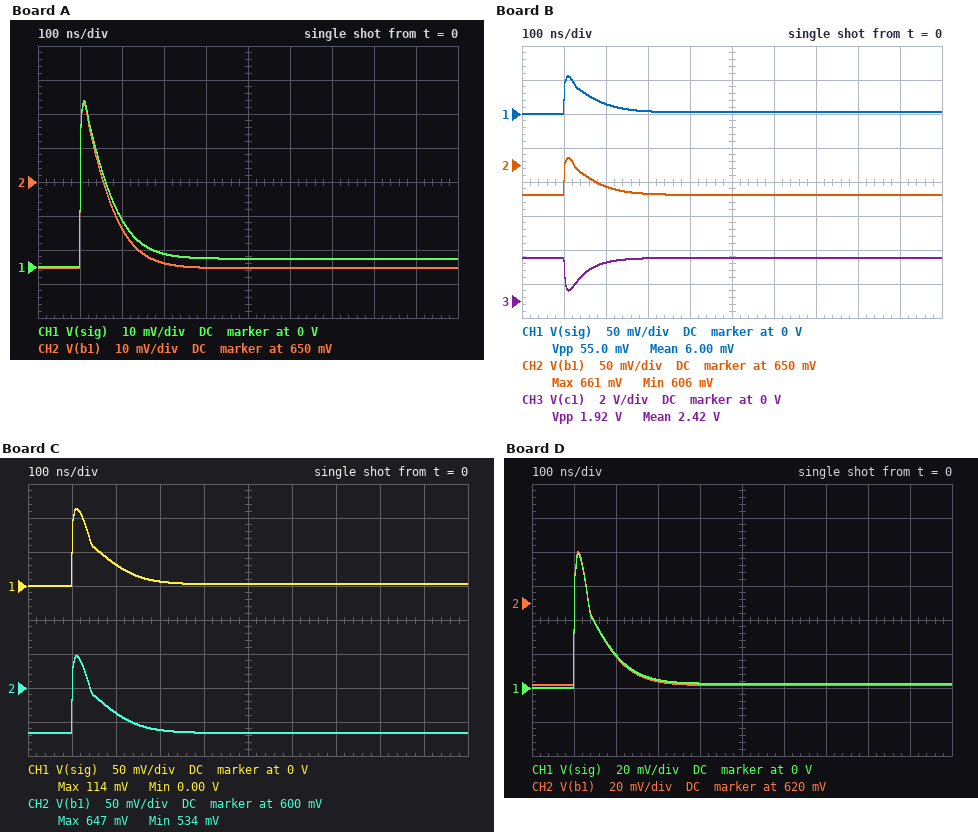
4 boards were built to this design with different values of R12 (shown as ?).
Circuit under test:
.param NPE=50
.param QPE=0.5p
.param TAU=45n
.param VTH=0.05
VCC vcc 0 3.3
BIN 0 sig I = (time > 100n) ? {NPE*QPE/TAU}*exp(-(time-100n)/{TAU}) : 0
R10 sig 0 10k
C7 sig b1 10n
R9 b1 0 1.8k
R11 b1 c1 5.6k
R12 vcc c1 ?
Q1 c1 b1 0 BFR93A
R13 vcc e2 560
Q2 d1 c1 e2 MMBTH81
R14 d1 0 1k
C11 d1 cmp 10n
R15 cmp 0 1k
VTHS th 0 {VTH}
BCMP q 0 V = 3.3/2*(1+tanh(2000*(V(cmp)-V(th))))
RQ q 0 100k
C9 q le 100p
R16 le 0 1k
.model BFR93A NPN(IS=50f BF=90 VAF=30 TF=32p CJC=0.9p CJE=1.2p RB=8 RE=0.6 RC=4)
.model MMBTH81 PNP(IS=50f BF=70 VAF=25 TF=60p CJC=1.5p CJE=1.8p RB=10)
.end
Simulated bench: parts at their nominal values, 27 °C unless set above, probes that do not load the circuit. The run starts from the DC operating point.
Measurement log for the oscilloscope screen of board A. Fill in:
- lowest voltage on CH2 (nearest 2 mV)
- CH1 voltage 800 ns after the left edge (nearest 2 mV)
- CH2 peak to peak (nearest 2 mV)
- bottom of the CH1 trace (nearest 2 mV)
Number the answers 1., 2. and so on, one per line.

1. 624 mV
2. 2 mV
3. 48 mV
4. 0 V
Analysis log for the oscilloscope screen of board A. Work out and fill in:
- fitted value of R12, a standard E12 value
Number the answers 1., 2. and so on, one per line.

1. 330 Ω
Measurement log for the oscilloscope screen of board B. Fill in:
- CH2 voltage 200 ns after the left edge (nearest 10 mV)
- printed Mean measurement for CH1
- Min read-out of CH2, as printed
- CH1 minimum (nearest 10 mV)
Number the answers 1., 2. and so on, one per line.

1. 620 mV
2. 6.00 mV
3. 606 mV
4. 0 V
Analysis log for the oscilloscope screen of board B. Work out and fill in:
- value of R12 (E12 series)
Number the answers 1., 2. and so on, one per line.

1. 680 Ω
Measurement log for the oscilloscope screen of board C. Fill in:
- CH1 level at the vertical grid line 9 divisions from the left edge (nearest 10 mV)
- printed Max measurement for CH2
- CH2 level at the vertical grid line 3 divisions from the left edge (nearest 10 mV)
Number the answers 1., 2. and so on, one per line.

1. 0 V
2. 647 mV
3. 540 mV
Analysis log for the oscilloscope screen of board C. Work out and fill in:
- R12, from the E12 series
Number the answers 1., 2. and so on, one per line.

1. 3.3 kΩ
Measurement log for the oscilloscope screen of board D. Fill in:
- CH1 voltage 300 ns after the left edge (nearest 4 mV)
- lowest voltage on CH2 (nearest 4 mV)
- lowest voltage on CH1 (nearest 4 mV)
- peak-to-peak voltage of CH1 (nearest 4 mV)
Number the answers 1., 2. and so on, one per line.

1. 4 mV
2. 572 mV
3. 0 V
4. 80 mV
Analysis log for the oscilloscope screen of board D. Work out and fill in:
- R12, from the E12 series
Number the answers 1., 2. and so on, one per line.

1. 1.8 kΩ
